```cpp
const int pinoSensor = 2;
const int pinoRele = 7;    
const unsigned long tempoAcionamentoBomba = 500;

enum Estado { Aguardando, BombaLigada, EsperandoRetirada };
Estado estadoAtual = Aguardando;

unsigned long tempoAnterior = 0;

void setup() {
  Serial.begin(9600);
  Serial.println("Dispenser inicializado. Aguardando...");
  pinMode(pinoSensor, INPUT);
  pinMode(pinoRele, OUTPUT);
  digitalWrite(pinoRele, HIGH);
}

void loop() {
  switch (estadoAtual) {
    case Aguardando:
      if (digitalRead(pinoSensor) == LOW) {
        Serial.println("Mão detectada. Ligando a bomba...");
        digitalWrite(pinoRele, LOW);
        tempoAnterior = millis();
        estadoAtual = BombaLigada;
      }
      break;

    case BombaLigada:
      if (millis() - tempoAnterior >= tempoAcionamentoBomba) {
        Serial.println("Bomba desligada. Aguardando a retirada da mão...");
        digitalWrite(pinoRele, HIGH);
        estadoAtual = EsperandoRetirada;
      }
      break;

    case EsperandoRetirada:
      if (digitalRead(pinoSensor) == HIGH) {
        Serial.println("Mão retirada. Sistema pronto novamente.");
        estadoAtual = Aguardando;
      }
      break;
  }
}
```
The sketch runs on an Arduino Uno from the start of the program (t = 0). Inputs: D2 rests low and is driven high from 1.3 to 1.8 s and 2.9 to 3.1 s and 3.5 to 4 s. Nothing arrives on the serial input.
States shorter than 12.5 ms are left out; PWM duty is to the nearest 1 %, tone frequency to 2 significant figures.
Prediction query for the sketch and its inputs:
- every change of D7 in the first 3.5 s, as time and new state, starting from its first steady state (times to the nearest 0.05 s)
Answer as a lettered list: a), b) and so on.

a) 0 s low; 0.5 s high; 1.8 s low; 2.3 s high; 3.1 s low
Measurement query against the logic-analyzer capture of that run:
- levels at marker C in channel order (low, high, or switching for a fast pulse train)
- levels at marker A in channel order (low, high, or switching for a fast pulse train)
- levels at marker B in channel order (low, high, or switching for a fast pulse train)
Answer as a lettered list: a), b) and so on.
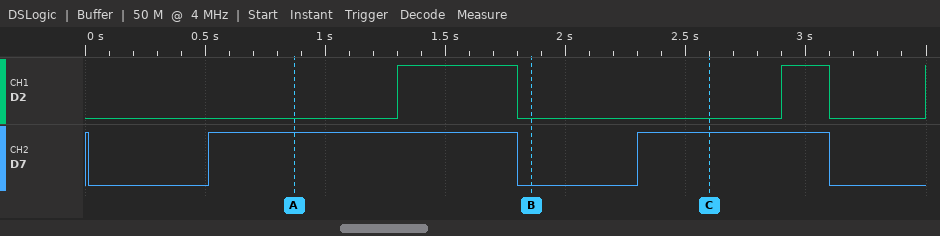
a) D2 low, D7 high
b) D2 low, D7 high
c) D2 low, D7 low
